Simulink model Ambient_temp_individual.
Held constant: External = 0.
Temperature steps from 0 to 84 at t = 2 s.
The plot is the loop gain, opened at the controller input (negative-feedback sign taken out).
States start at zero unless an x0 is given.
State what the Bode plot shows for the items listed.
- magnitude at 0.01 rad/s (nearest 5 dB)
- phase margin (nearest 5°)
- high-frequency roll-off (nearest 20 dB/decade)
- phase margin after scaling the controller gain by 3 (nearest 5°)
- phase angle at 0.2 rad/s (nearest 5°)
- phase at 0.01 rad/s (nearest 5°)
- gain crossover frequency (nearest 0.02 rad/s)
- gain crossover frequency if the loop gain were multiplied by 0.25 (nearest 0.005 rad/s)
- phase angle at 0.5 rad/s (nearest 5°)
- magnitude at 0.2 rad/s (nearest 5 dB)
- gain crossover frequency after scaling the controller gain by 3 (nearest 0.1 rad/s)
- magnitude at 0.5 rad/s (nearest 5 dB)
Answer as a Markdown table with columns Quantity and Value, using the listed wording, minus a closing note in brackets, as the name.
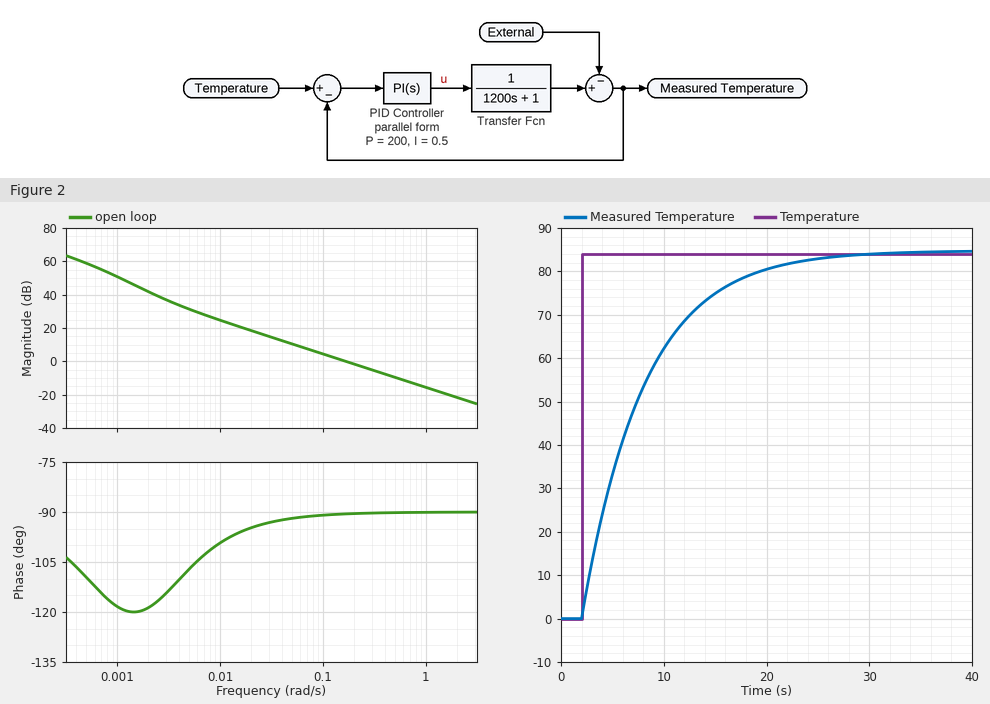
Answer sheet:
| Quantity | Value |
|---|---|
| magnitude at 0.01 rad/s | 25 dB |
| phase margin | 90° |
| high-frequency roll-off | -20 dB/decade |
| phase margin after scaling the controller gain by 3 | 90° |
| phase angle at 0.2 rad/s | -90° |
| phase at 0.01 rad/s | -100° |
| gain crossover frequency | 0.16 rad/s |
| gain crossover frequency if the loop gain were multiplied by 0.25 | 0.040 rad/s |
| phase angle at 0.5 rad/s | -90° |
| magnitude at 0.2 rad/s | 0 dB |
| gain crossover frequency after scaling the controller gain by 3 | 0.5 rad/s |
| magnitude at 0.5 rad/s | -10 dB |
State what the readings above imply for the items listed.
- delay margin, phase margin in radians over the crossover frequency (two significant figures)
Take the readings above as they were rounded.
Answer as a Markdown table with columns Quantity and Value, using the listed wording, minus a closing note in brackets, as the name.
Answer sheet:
| Quantity | Value |
|---|---|
| delay margin, phase margin in radians over the crossover frequency | 9.8 s |
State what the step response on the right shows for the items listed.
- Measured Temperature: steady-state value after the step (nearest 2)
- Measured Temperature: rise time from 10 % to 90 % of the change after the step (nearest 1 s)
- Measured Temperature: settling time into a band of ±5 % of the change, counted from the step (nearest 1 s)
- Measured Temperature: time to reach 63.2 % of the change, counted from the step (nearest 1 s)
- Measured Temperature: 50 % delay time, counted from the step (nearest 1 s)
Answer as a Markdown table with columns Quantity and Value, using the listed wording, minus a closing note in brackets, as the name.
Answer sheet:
| Quantity | Value |
|---|---|
| Measured Temperature: steady-state value after the step | 84 |
| Measured Temperature: rise time from 10 % to 90 % of the change after the step | 13 s |
| Measured Temperature: settling time into a band of ±5 % of the change, counted from the step | 18 s |
| Measured Temperature: time to reach 63.2 % of the change, counted from the step | 6 s |
| Measured Temperature: 50 % delay time, counted from the step | 4 s |
